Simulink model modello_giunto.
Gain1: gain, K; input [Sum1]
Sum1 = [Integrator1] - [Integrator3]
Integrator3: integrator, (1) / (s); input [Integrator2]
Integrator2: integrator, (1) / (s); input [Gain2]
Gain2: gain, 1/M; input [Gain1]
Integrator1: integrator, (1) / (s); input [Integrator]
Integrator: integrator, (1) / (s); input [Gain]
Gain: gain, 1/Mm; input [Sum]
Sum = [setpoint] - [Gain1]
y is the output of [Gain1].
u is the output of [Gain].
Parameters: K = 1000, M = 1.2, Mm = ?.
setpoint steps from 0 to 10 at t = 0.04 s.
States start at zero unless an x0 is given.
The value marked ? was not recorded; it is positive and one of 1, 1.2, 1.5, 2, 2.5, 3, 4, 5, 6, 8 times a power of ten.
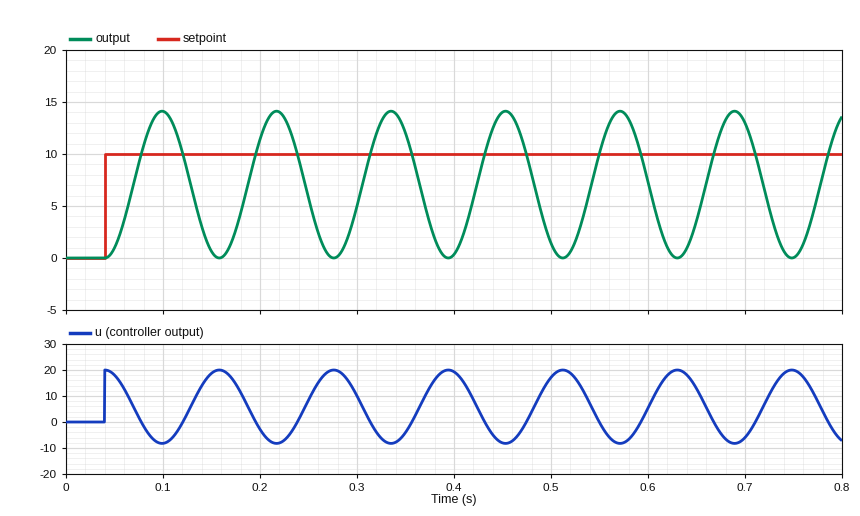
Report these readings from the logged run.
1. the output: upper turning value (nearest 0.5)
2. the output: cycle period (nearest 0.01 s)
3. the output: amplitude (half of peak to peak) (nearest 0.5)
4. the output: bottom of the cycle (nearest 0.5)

14.0
0.12 s
7.0
0.0
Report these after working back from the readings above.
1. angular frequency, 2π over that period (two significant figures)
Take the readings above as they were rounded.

52 rad/s
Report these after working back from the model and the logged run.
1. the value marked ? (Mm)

0.5
